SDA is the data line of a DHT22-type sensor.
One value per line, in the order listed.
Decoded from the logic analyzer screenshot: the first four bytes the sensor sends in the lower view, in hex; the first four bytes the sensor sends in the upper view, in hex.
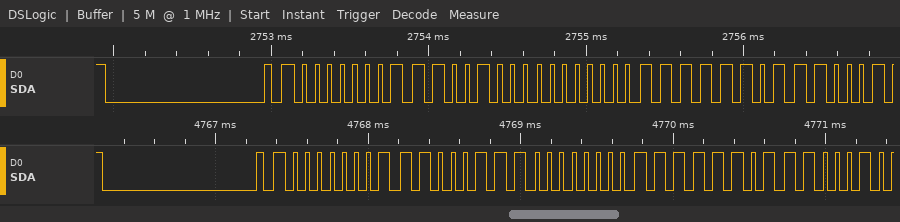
01, C7, 00, FD
01, C8, 00, FD
